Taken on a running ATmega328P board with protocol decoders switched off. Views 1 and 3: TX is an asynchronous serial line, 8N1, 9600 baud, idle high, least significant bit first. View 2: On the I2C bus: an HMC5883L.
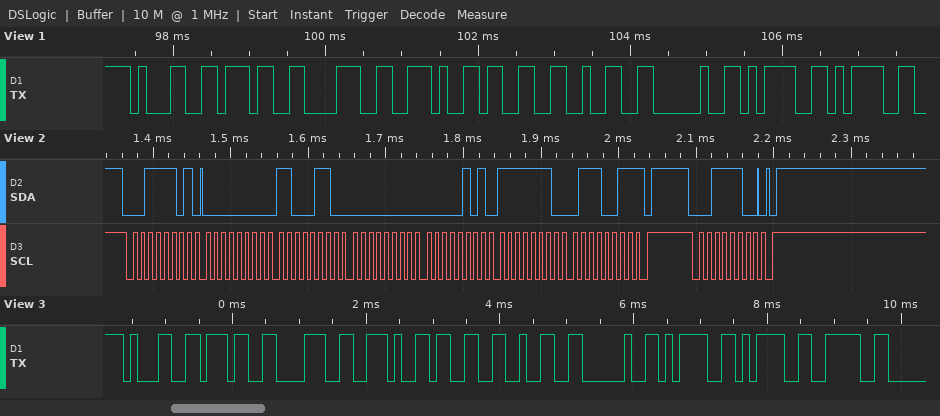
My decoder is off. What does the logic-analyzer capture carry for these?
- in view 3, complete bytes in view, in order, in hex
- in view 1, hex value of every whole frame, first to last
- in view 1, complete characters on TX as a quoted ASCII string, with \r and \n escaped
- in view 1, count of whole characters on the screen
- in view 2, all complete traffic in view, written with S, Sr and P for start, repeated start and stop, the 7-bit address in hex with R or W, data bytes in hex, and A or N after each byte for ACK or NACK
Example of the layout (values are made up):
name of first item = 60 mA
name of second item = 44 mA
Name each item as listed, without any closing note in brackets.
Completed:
in view 3, complete bytes in view, in order, in hex = 31 37 38 2E 33 32 20 3D 3D 3E
in view 1, hex value of every whole frame, first to last = 31 37 38 2E 33 32 20 3D 3D
in view 1, complete characters on TX as a quoted ASCII string, with \r and \n escaped = "178.32 =="
in view 1, count of whole characters on the screen = 9
in view 2, all complete traffic in view, written with S, Sr and P for start, repeated start and stop, the 7-bit address in hex with R or W, data bytes in hex, and A or N after each byte for ACK or NACK = S 1ER A 00 A C6 A 00 A 05 A FE A 73 N P S 1EW A P
